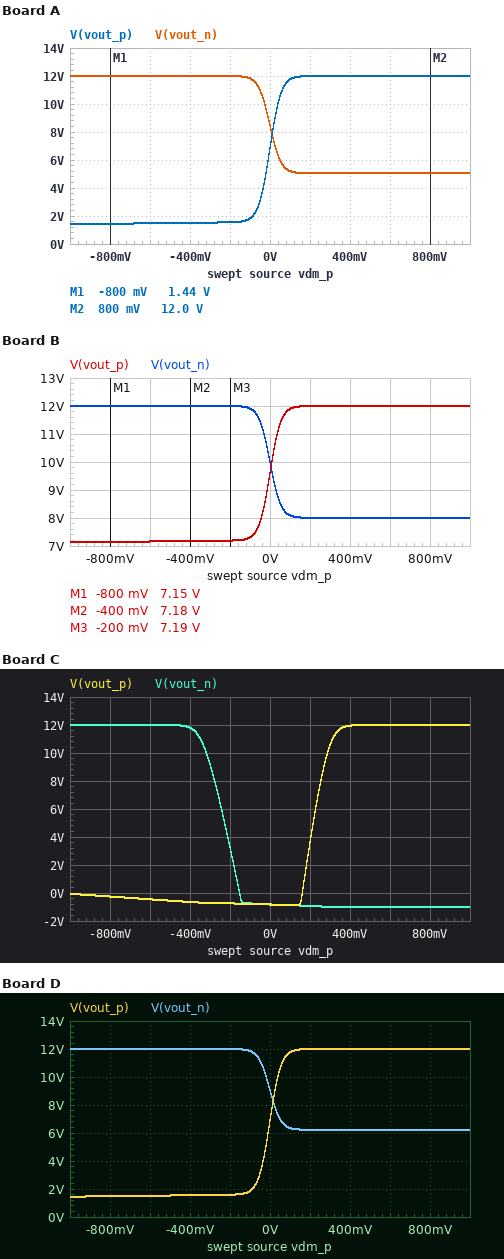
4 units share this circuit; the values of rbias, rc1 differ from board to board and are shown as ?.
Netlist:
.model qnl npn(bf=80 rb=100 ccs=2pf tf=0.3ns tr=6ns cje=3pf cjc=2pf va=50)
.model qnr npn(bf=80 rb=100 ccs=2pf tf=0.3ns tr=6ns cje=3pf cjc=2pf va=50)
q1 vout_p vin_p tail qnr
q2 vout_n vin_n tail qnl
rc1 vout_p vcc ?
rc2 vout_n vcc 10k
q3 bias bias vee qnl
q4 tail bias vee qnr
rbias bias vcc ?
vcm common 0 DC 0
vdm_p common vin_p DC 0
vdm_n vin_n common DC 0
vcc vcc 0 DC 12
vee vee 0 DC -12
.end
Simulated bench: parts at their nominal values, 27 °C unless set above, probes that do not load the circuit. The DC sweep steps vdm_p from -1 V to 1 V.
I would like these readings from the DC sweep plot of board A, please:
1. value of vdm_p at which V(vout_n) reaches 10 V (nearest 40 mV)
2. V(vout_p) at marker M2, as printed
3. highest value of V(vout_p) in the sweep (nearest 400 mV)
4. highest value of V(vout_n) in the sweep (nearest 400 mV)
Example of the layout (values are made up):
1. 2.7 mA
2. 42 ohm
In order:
1. -40 mV
2. 12.0 V
3. 12.0 V
4. 12.0 V
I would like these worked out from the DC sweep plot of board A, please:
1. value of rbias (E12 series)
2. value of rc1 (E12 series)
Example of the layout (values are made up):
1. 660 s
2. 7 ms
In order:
1. 39 kΩ
2. 15 kΩ
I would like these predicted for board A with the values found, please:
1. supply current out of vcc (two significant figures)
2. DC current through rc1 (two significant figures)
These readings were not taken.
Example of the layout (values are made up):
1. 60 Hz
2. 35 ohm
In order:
1. 1.3 mA
2. 340 µA
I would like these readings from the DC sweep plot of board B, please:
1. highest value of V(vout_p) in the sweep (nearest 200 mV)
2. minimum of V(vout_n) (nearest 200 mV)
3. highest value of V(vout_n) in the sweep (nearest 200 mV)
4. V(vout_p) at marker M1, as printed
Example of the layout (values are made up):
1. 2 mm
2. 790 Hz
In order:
1. 12.0 V
2. 8.0 V
3. 12.0 V
4. 7.15 V
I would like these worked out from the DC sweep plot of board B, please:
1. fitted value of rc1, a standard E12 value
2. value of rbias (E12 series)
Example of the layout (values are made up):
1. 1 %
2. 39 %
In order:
1. 12 kΩ
2. 68 kΩ
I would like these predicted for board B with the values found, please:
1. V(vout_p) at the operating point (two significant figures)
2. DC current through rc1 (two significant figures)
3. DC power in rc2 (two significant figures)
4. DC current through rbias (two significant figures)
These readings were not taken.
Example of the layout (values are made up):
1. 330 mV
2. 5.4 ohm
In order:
1. 9.6 V
2. 200 µA
3. 400 µW
4. 340 µA
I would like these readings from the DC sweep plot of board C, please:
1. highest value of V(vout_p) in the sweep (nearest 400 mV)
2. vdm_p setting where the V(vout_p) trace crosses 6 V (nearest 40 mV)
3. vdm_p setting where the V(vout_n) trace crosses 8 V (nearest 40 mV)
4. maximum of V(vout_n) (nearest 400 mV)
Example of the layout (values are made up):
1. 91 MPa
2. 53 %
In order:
1. 12.0 V
2. 240 mV
3. -280 mV
4. 12.0 V
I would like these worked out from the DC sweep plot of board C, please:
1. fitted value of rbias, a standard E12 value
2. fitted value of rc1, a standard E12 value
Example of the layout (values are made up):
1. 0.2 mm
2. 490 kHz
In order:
1. 8.2 kΩ
2. 15 kΩ
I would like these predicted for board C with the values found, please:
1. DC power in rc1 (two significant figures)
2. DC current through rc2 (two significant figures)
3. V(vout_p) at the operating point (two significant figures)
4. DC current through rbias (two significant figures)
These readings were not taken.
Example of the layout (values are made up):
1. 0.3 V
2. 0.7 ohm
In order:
1. 11 mW
2. 1.3 mA
3. -820 mV
4. 2.8 mA
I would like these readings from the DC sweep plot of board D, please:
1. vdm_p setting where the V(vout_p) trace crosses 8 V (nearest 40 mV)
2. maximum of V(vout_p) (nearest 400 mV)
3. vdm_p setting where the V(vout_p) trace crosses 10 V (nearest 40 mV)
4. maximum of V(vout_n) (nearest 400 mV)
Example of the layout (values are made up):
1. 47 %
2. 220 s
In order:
1. 0 V
2. 12.0 V
3. 40 mV
4. 12.0 V
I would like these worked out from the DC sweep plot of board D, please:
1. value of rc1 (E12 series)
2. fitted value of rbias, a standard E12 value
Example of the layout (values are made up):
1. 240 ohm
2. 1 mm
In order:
1. 18 kΩ
2. 47 kΩ
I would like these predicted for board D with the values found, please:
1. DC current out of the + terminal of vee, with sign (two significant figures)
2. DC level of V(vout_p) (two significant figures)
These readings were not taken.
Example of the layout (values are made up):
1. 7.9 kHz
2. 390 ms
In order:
1. -1.1 mA
2. 6.9 V
